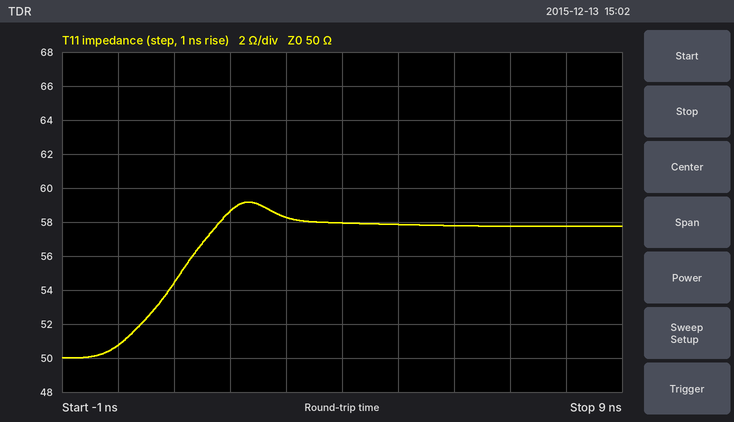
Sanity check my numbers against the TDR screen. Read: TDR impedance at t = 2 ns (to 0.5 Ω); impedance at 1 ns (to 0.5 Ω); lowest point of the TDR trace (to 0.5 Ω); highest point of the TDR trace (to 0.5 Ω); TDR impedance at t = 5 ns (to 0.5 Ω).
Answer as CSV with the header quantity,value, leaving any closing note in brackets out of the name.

quantity,value
TDR impedance at t = 2 ns,58.5 Ω
impedance at 1 ns,54.5 Ω
lowest point of the TDR trace,50.0 Ω
highest point of the TDR trace,59.0 Ω
TDR impedance at t = 5 ns,58.0 Ω
